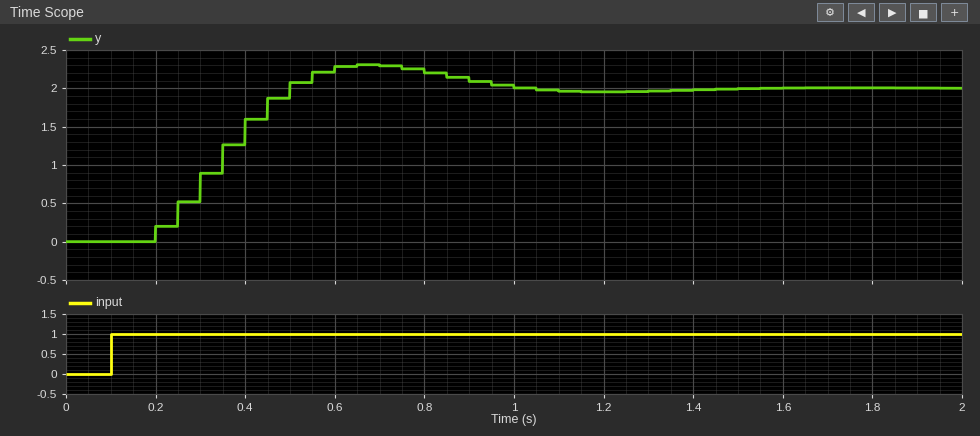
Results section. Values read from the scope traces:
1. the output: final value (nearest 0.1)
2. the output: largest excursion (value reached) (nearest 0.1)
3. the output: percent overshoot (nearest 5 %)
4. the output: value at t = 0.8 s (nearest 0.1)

2.0
2.3
15 %
2.2
